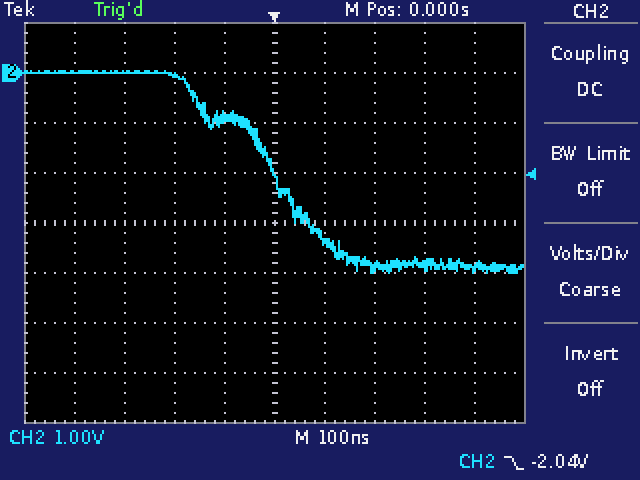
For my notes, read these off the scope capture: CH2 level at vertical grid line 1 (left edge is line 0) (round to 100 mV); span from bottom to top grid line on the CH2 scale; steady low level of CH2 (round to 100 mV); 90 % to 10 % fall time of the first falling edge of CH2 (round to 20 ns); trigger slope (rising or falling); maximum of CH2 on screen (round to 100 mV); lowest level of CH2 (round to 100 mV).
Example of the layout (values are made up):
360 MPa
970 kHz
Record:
0.0 V
8 V
-3.9 V
280 ns
falling
0.0 V
-4.0 V
